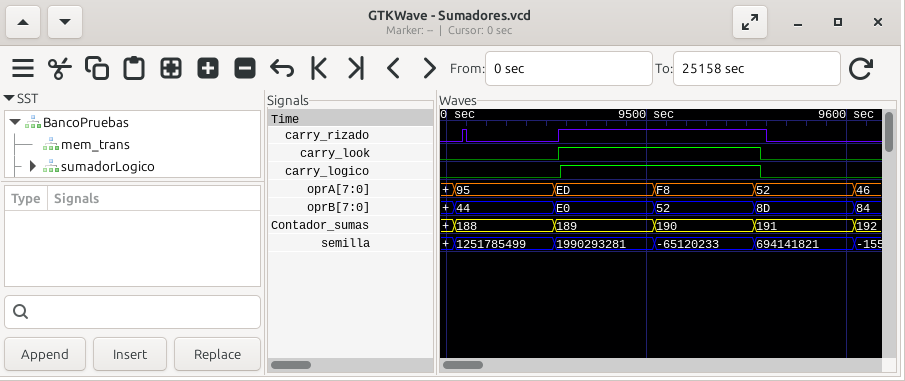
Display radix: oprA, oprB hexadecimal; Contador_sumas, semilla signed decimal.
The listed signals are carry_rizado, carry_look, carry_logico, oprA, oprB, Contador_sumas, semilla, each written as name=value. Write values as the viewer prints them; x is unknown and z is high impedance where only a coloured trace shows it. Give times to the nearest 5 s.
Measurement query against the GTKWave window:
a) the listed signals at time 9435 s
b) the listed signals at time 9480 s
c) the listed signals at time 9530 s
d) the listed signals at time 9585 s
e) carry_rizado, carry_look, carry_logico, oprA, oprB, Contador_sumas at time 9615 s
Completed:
carry_rizado=0, carry_look=0, carry_logico=0, oprA=95, oprB=44, Contador_sumas=188, semilla=1251785499
carry_rizado=1, carry_look=1, carry_logico=1, oprA=ED, oprB=E0, Contador_sumas=189, semilla=1990293281
carry_rizado=1, carry_look=1, carry_logico=1, oprA=F8, oprB=52, Contador_sumas=190, semilla=-65120233
carry_rizado=0, carry_look=0, carry_logico=0, oprA=52, oprB=8D, Contador_sumas=191, semilla=694141821
carry_rizado=0, carry_look=0, carry_logico=0, oprA=46, oprB=84, Contador_sumas=192
